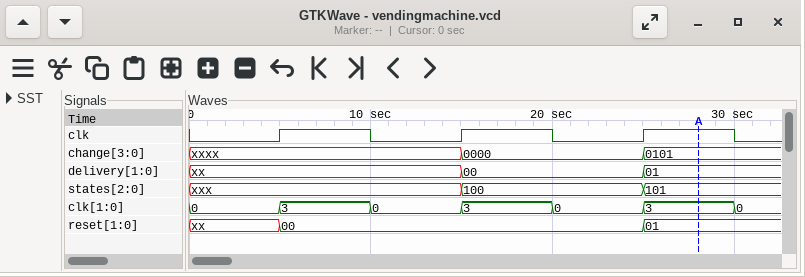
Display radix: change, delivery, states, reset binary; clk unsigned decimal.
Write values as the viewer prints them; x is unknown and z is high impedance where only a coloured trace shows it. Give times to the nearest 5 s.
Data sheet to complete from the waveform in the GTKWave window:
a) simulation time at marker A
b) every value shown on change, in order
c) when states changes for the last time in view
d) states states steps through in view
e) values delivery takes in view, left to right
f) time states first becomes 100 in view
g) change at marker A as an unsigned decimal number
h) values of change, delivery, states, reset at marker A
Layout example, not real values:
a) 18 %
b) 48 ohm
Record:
a) 30 s
b) xxxx, 0000, 0101
c) 25 s
d) xxx, 100, 101
e) xx, 00, 01
f) 15 s
g) 5
h) change=0101, delivery=01, states=101, reset=01
